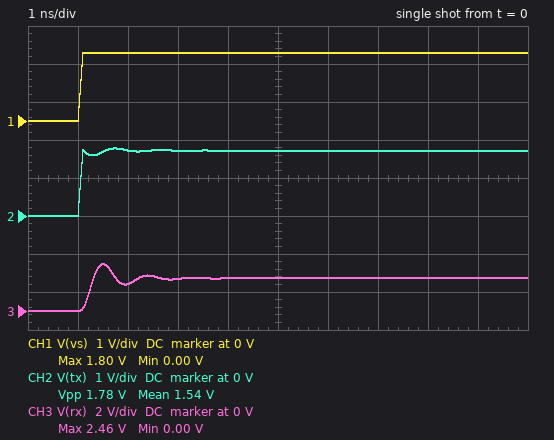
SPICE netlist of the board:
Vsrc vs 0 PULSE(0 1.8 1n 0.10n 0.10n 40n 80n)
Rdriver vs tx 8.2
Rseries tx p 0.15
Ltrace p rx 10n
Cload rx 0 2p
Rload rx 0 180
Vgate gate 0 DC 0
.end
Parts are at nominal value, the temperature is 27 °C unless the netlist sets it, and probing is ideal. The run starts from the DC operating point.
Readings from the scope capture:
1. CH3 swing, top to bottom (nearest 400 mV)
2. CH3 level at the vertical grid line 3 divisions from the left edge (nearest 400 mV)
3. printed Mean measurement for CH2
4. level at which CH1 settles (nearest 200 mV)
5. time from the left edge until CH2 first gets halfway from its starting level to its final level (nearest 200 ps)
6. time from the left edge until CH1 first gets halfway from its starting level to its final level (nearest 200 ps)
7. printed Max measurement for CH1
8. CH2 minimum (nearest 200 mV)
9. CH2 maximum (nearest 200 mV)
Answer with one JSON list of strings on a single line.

["2.4 V", "1.6 V", "1.54 V", "1.8 V", "1.0 ns", "1.0 ns", "1.80 V", "0 V", "1.8 V"]
